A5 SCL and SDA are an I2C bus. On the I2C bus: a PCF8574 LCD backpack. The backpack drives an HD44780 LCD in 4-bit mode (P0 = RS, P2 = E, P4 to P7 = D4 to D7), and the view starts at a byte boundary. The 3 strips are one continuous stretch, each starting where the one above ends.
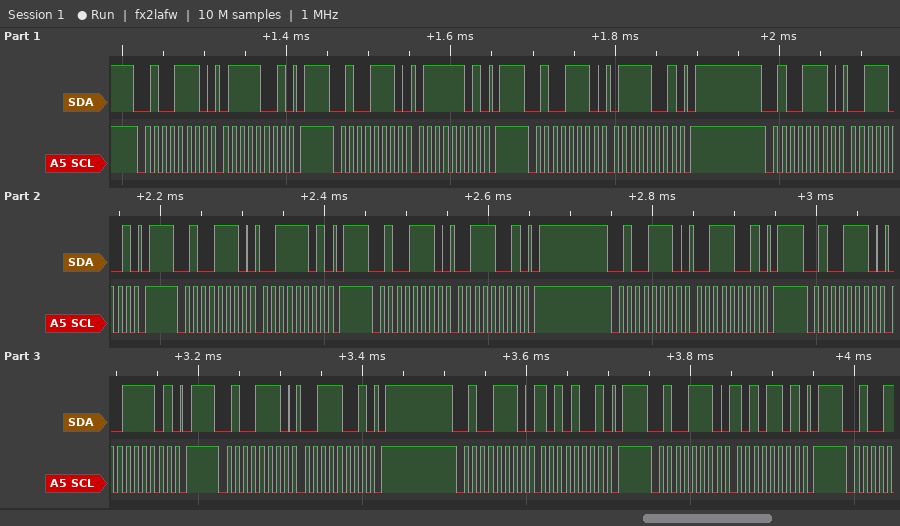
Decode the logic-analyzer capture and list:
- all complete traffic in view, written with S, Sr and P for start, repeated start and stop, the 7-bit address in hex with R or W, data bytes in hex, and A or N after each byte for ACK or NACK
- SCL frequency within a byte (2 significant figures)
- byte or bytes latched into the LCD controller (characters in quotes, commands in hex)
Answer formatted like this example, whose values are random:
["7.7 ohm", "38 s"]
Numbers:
["S 27W A 79 A P S 27W A 7D A P S 27W A 79 A P S 27W A 39 A P S 27W A 3D A P S 27W A 39 A P S 27W A 39 A P S 27W A 3D A P S 27W A 39 A P S 27W A A9 A P S 27W A AD A P", "100 kHz", "'s'"]
